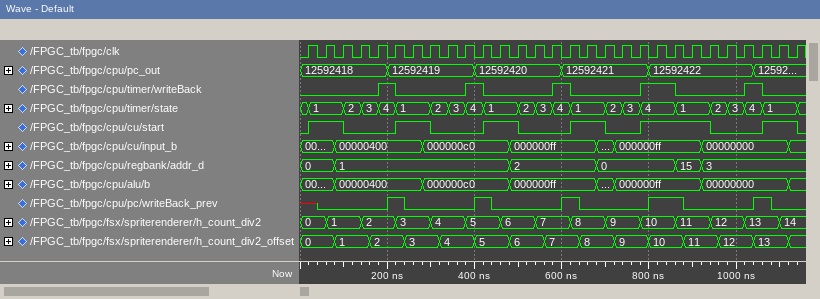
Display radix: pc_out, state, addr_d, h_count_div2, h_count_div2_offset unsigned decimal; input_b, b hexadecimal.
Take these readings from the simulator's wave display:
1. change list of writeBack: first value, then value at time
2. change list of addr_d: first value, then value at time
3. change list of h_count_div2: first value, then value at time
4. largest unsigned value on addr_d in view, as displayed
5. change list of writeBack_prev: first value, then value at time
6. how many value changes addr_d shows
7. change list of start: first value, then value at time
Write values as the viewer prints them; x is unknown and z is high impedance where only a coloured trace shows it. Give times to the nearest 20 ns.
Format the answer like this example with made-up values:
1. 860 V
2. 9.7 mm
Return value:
1. 0, 1 at 180 ns, 0 at 220 ns, 1 at 380 ns, 0 at 420 ns, 1 at 580 ns, 0 at 620 ns, 1 at 780 ns, 0 at 860 ns, 1 at 1020 ns, 0 at 1060 ns
2. 0, 1 at 80 ns, 2 at 480 ns, 0 at 680 ns, 15 at 860 ns, 3 at 920 ns
3. 0, 1 at 60 ns, 2 at 140 ns, 3 at 220 ns, 4 at 300 ns, 5 at 380 ns, 6 at 460 ns, 7 at 540 ns, 8 at 620 ns, 9 at 700 ns, 10 at 780 ns, 11 at 860 ns, 12 at 940 ns, 13 at 1020 ns, 14 at 1100 ns
4. 15
5. x, 0 at 40 ns, 1 at 200 ns, 0 at 240 ns, 1 at 400 ns, 0 at 440 ns, 1 at 600 ns, 0 at 640 ns, 1 at 800 ns, 0 at 880 ns, 1 at 1040 ns, 0 at 1080 ns
6. 5
7. 0, 1 at 20 ns, 0 at 100 ns, 1 at 220 ns, 0 at 300 ns, 1 at 420 ns, 0 at 500 ns, 1 at 620 ns, 0 at 700 ns, 1 at 780 ns, 0 at 940 ns, 1 at 1060 ns, 0 at 1140 ns
